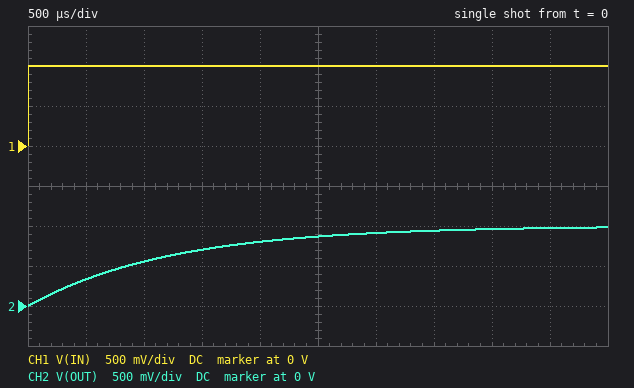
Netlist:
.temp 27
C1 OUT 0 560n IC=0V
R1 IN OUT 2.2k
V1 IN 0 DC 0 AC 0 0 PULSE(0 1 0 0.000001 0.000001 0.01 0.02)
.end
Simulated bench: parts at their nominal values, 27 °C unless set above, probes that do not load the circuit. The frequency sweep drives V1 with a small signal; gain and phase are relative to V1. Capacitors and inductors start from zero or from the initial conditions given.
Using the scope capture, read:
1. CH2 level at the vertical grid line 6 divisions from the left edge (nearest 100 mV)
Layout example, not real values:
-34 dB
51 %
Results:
900 mV
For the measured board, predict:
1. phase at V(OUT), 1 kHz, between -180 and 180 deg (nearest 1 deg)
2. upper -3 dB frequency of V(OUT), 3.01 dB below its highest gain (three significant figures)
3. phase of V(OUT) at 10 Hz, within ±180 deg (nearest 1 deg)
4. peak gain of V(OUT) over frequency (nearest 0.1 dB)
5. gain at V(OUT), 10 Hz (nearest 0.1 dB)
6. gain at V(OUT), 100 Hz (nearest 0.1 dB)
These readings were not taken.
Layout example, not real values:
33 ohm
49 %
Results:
-83 deg
129 Hz
-4 deg
0 dB
0 dB
-2.0 dB
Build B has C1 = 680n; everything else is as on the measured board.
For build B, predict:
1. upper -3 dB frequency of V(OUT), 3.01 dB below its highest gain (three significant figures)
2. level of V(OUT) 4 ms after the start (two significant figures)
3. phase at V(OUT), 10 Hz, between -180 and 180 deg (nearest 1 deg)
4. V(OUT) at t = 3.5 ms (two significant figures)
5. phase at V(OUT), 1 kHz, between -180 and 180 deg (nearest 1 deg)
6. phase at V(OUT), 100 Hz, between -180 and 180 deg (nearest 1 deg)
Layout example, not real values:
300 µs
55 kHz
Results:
106 Hz
930 mV
-5 deg
900 mV
-84 deg
-43 deg
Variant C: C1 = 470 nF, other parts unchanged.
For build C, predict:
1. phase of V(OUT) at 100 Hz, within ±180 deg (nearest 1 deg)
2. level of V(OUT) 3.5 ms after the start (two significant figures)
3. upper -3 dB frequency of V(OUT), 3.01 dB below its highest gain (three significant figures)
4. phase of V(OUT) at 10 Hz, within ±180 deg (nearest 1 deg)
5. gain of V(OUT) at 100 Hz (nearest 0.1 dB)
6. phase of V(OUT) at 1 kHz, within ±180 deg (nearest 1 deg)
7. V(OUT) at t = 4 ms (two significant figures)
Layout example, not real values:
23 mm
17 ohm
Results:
-33 deg
970 mV
154 Hz
-4 deg
-1.5 dB
-81 deg
980 mV
